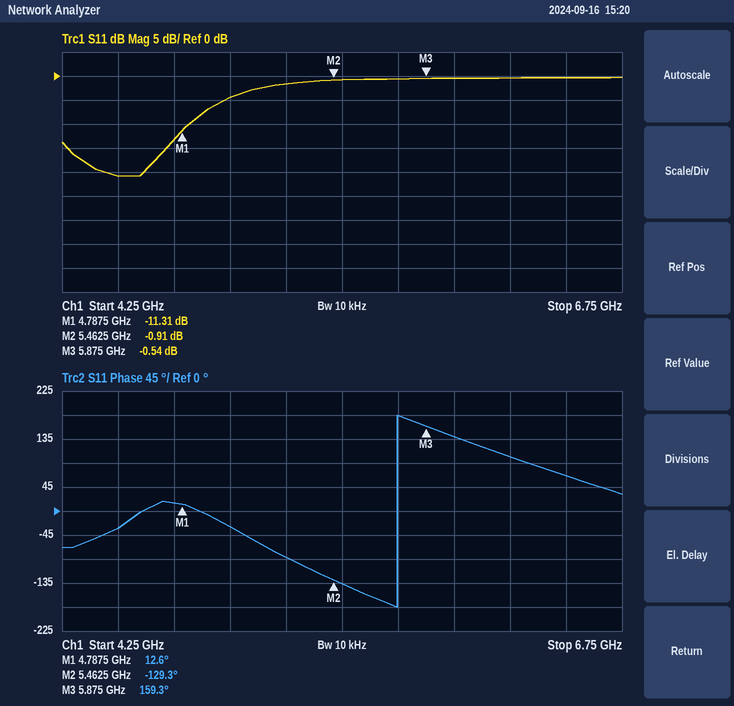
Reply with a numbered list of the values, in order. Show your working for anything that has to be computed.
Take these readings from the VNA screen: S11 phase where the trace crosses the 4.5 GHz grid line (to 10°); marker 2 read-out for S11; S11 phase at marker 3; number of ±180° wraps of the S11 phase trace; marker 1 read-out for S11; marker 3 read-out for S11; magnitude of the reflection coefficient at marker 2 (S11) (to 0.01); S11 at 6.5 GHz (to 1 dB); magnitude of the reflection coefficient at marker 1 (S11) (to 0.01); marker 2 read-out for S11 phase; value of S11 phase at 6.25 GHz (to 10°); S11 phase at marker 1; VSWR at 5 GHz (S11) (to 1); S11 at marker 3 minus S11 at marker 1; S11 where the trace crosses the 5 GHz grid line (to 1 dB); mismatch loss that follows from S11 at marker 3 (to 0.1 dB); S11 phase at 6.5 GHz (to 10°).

1. -30°
2. -0.91 dB
3. 159.3°
4. 1
5. -11.31 dB
6. -0.54 dB
7. 10^(-0.91/20) ≈ 0.90
8. 0 dB
9. 10^(-11.31/20) ≈ 0.27
10. -129.3°
11. 100°
12. 12.6°
13. |Γ| = 10^(-4/20) = 0.6310; VSWR = (1 + 0.6310)/(1 − 0.6310) ≈ 4
14. -0.54 − (-11.31) = 10.77 dB
15. -4 dB
16. −10 log10(1 − 10^(-0.54/10)) ≈ 9.3 dB
17. 70°
